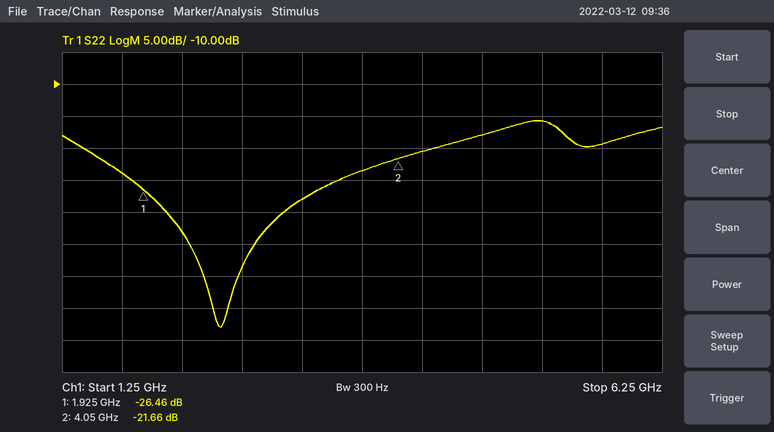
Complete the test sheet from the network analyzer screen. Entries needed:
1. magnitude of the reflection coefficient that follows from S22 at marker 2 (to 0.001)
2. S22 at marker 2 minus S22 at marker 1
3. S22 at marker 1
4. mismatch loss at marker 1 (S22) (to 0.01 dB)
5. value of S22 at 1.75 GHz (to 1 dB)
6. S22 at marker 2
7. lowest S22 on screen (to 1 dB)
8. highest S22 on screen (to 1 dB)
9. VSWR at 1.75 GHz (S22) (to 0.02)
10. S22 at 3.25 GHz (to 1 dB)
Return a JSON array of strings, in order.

["0.083", "4.80 dB", "-26.46 dB", "0.01 dB", "-24 dB", "-21.66 dB", "-48 dB", "-16 dB", "1.14", "-28 dB"]
